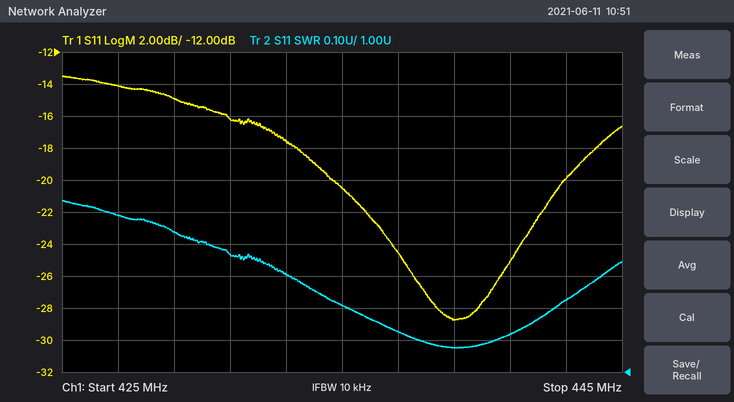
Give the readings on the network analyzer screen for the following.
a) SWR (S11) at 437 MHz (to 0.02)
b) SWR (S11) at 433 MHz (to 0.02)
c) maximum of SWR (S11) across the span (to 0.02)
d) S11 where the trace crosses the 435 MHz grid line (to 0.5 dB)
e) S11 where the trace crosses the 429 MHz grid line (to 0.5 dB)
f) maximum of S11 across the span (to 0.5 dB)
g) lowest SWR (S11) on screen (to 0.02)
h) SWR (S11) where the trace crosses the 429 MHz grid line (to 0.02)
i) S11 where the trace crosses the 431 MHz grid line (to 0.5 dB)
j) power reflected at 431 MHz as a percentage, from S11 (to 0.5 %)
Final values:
1.12
1.30
1.54
-20.5 dB
-15.0 dB
-13.5 dB
1.08
1.44
-16.0 dB
2.5 %
